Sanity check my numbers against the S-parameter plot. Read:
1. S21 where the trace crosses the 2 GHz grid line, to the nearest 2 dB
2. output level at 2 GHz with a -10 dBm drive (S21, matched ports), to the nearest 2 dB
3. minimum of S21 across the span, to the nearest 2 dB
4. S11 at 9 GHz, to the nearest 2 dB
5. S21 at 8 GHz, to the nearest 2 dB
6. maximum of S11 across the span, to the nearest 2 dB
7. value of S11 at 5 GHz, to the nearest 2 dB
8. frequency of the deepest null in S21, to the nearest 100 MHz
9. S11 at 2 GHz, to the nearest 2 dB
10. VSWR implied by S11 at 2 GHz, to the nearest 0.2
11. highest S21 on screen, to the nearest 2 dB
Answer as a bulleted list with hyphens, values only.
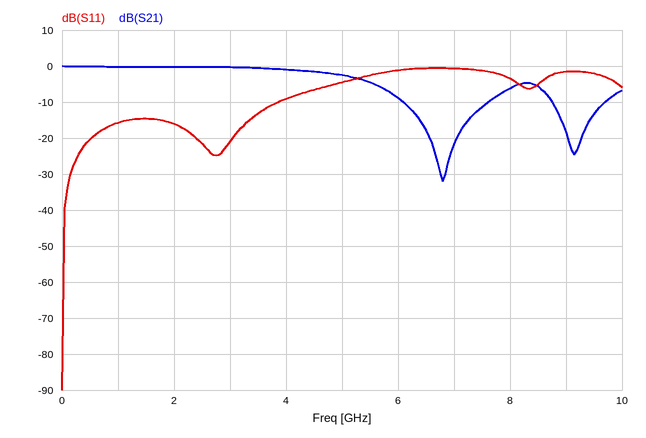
- 0 dB
- -10 dBm
- -32 dB
- -2 dB
- -6 dB
- 0 dB
- -4 dB
- 6.8 GHz
- -16 dB
- 1.4
- 0 dB
